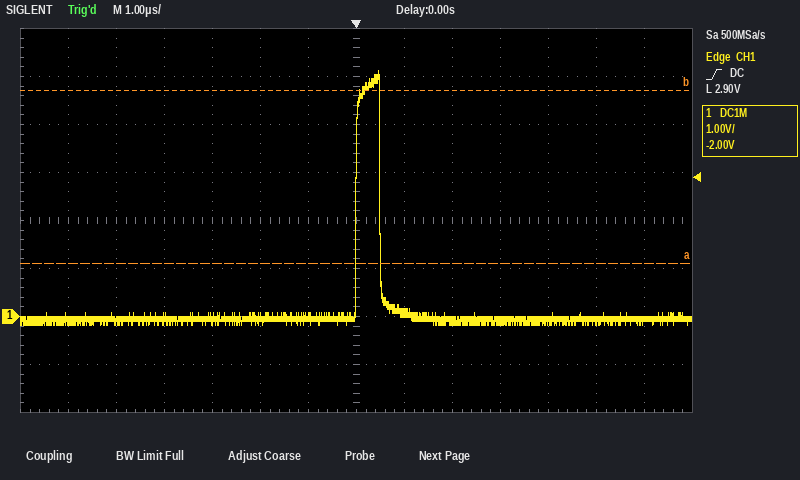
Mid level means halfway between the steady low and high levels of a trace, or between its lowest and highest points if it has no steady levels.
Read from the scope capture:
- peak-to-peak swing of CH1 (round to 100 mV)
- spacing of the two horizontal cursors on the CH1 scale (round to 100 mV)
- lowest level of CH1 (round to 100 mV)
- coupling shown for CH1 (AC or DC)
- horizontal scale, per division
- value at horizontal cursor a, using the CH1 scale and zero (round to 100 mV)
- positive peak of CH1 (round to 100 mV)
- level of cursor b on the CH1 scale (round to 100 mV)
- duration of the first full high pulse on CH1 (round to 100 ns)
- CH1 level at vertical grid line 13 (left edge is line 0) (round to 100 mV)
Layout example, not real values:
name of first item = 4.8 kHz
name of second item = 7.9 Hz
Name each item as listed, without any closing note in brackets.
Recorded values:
peak-to-peak swing of CH1 = 5.3 V
spacing of the two horizontal cursors on the CH1 scale = 3.6 V
lowest level of CH1 = -200 mV
coupling shown for CH1 = DC
horizontal scale, per division = 1 µs
value at horizontal cursor a, using the CH1 scale and zero = 1.1 V
positive peak of CH1 = 5.1 V
level of cursor b on the CH1 scale = 4.7 V
duration of the first full high pulse on CH1 = 500 ns
CH1 level at vertical grid line 13 (left edge is line 0) = -100 mV
